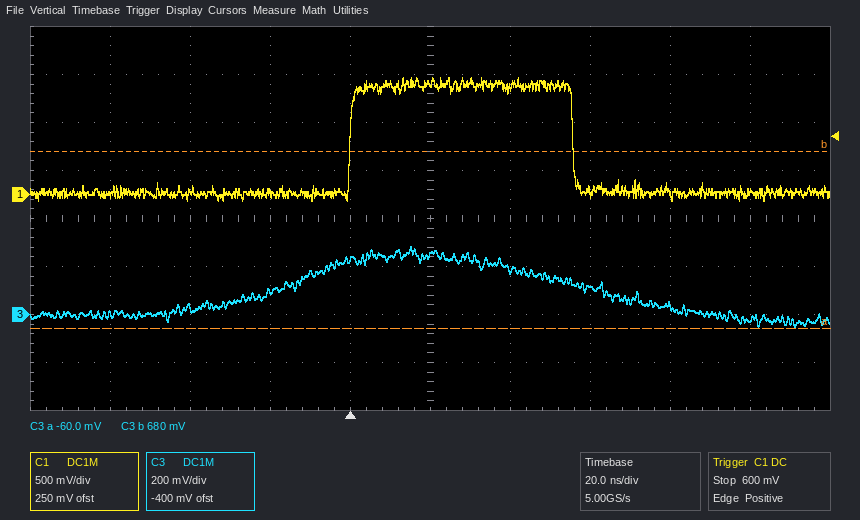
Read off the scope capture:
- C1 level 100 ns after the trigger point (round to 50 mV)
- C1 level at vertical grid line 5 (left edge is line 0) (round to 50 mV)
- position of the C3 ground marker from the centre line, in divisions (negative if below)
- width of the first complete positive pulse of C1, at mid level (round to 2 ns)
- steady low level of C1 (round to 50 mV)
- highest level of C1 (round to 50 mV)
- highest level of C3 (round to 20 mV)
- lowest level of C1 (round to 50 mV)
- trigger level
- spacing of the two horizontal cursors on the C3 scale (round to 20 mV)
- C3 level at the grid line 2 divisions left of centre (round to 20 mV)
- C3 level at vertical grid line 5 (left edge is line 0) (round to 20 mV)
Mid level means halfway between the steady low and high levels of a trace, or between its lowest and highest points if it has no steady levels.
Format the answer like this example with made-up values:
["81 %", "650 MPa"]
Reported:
["0 mV", "1.15 V", "-2.0 div", "56 ns", "0 mV", "1.20 V", "280 mV", "-50 mV", "600 mV", "740 mV", "100 mV", "240 mV"]
